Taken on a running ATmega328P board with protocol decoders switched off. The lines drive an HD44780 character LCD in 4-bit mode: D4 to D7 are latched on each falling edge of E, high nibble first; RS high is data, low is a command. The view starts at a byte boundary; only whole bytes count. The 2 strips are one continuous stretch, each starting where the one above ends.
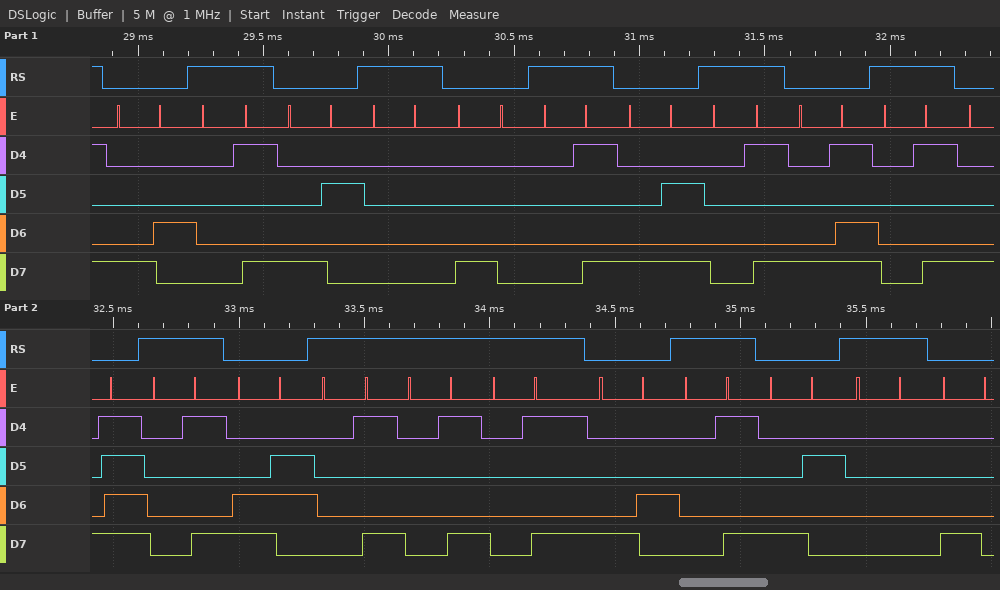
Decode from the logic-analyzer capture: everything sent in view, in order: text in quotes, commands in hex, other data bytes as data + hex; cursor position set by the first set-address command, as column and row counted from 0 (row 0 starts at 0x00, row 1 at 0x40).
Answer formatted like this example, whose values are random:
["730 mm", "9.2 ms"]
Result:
["0x84 data 09 0x82 data 00 0x80 data 09 0x8A data 09 0x8D data 09 0x8F data 09 0xC6 data 09 09 09 0x84 data 09 0x82 data 00 0x80", "column 4, row 0"]
